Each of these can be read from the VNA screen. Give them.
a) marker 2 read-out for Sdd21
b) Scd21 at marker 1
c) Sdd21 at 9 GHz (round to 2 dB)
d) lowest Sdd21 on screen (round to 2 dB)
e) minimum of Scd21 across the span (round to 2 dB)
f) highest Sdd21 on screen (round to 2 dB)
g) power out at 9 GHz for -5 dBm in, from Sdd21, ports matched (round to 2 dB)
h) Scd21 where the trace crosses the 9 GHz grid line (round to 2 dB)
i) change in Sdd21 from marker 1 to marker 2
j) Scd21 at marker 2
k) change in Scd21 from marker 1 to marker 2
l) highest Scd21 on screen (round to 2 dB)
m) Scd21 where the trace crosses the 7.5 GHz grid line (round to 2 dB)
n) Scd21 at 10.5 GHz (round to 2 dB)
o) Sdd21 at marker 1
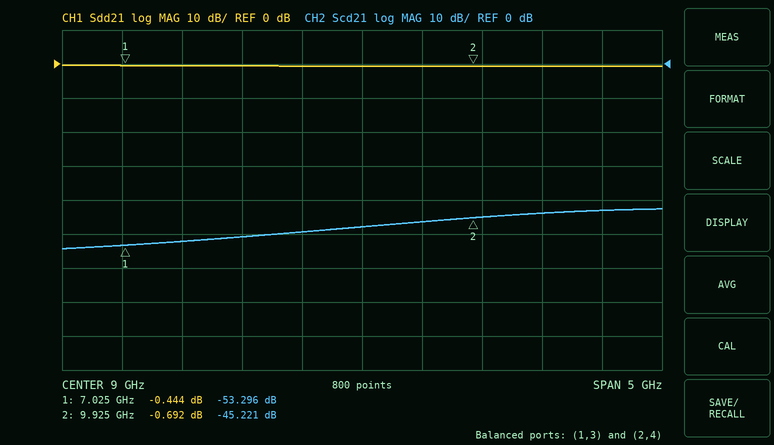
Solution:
-0.692 dB
-53.296 dB
0 dB
0 dB
-54 dB
0 dB
-6 dBm
-48 dB
-0.248 dB
-45.221 dB
8.075 dB
-42 dB
-52 dB
-44 dB
-0.444 dB
